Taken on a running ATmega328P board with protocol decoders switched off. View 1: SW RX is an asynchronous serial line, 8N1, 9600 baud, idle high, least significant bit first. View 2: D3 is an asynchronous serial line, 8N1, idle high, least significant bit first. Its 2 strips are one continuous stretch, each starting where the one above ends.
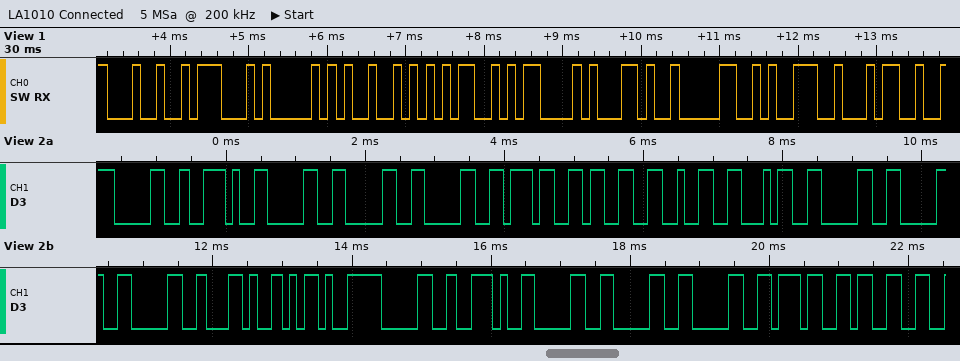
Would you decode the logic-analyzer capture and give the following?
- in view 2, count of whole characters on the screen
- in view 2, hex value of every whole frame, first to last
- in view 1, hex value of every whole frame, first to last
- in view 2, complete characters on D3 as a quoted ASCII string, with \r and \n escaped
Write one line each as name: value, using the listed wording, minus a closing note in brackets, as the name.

in view 2, count of whole characters on the screen: 21
in view 2, hex value of every whole frame, first to last: 30 2E 30 30 30 37 33 32 34 30 30 30 2C 2D 30 2E 30 30 30 37 33
in view 1, hex value of every whole frame, first to last: 0x24 0x47 0x50 0x52 0x4D 0x43 0x2C 0x30 0x39 0x34
in view 2, complete characters on D3 as a quoted ASCII string, with \r and \n escaped: "0.0007324000,-0.00073"
